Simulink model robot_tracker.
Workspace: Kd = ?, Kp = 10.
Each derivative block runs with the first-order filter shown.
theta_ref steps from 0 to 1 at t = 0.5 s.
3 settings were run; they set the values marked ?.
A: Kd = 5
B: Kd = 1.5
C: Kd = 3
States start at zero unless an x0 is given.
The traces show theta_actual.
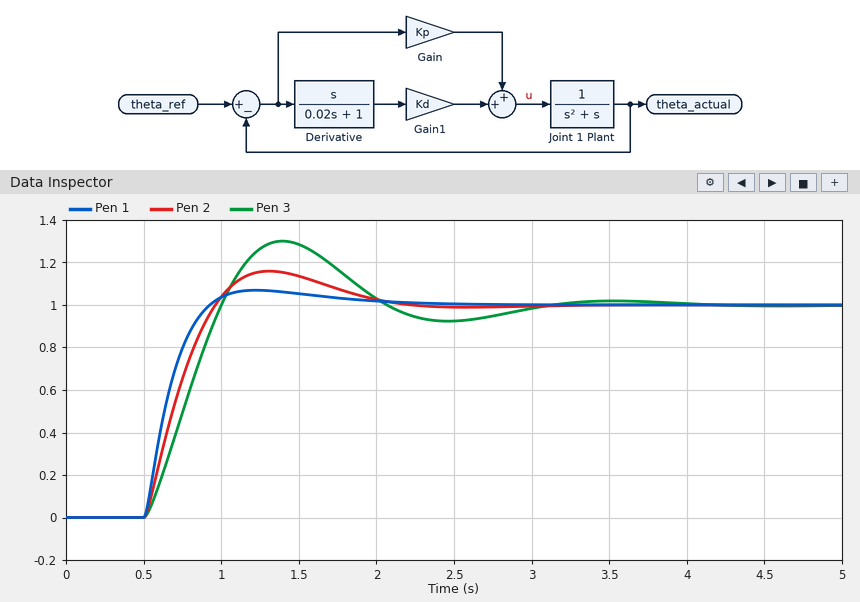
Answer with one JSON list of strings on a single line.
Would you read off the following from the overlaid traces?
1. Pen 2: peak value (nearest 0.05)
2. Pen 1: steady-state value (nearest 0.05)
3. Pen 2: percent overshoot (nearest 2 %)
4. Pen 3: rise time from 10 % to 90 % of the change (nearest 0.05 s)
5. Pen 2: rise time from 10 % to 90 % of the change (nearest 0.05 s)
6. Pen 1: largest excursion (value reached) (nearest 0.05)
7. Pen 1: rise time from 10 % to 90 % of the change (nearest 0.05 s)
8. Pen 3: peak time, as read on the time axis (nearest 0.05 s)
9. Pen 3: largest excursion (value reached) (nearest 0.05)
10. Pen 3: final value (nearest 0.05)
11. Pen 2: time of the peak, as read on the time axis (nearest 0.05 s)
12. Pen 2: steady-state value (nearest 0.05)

["1.15", "1.00", "16 %", "0.35 s", "0.35 s", "1.05", "0.30 s", "1.40 s", "1.30", "1.00", "1.30 s", "1.00"]
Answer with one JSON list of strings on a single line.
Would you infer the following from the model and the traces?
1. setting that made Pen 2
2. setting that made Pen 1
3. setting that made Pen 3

["C", "A", "B"]
